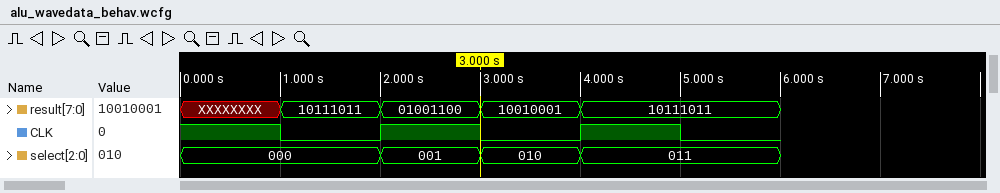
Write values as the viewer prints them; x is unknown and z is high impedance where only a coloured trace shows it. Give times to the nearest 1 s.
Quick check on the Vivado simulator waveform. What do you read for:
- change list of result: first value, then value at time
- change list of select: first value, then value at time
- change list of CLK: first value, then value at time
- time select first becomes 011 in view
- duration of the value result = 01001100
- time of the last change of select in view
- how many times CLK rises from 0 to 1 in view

XXXXXXXX, 10111011 at 1 s, 01001100 at 2 s, 10010001 at 3 s, 10111011 at 4 s
000, 001 at 2 s, 010 at 3 s, 011 at 4 s
1, 0 at 1 s, 1 at 2 s, 0 at 3 s, 1 at 4 s, 0 at 5 s
4 s
1 s
4 s
2
